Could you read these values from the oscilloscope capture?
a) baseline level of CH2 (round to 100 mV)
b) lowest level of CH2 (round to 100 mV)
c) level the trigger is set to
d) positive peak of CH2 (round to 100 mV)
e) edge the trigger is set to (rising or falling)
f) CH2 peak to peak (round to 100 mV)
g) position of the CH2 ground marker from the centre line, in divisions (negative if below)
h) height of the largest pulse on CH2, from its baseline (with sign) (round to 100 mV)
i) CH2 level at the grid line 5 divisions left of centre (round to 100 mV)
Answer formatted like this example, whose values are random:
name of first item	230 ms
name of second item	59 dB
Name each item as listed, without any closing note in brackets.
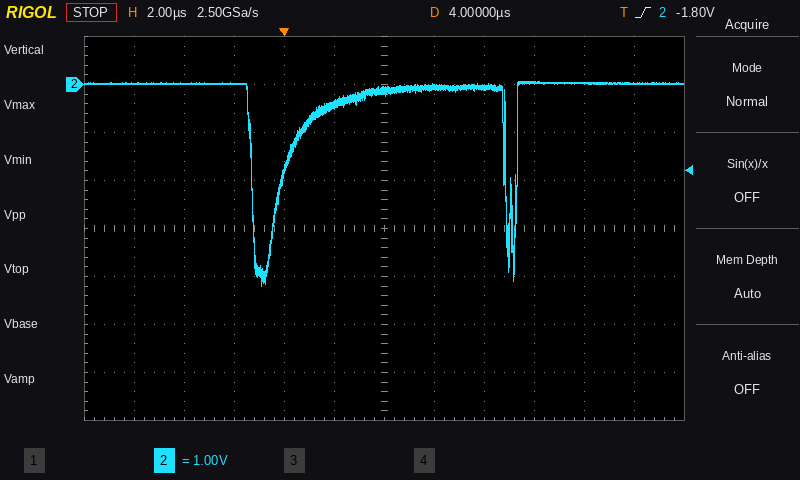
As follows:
baseline level of CH2	0.0 V
lowest level of CH2	-4.2 V
level the trigger is set to	-1.80 V
positive peak of CH2	100 mV
edge the trigger is set to	rising
CH2 peak to peak	4.3 V
position of the CH2 ground marker from the centre line, in divisions	+3.0 div
height of the largest pulse on CH2, from its baseline (with sign)	-4.2 V
CH2 level at the grid line 5 divisions left of centre	0.0 V
